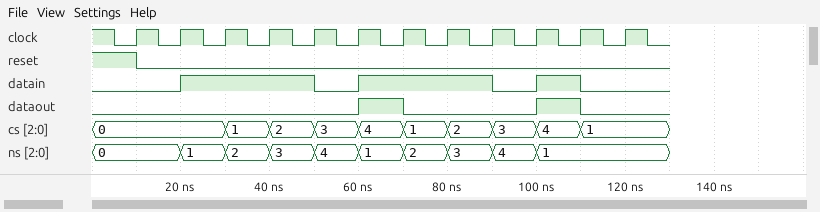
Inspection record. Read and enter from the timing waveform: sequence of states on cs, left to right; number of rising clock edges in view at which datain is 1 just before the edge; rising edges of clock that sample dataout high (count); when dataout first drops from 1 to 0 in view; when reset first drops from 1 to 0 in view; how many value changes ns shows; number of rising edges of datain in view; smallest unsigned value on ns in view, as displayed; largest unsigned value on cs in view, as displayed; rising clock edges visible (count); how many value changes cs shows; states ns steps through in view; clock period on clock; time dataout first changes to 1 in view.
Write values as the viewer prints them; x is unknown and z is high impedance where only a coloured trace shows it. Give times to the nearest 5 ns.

0, 1, 2, 3, 4, 1, 2, 3, 4, 1
7
2
70 ns
10 ns
9
3
0
4
12
9
0, 1, 2, 3, 4, 1, 2, 3, 4, 1
10 ns
60 ns
